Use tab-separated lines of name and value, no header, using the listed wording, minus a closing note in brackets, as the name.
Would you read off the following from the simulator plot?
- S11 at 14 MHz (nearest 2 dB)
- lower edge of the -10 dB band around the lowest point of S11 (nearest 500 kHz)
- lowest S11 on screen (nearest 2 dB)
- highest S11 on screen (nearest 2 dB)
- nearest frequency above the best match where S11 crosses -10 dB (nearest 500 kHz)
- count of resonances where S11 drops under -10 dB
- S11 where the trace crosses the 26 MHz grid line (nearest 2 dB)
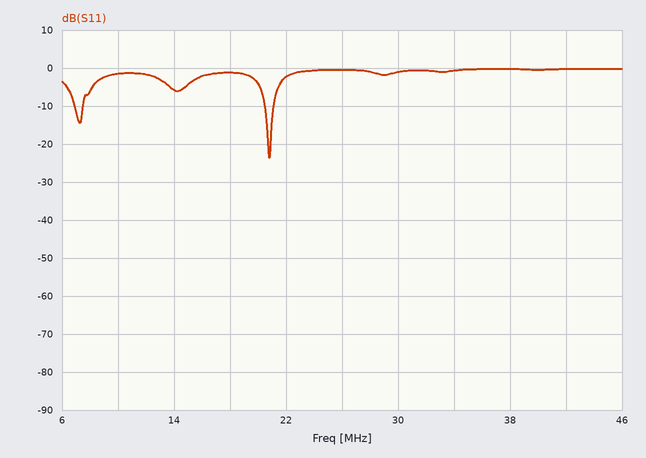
S11 at 14 MHz	-6 dB
lower edge of the -10 dB band around the lowest point of S11	20.5 MHz
lowest S11 on screen	-24 dB
highest S11 on screen	0 dB
nearest frequency above the best match where S11 crosses -10 dB	21.0 MHz
count of resonances where S11 drops under -10 dB	2
S11 where the trace crosses the 26 MHz grid line	0 dB
